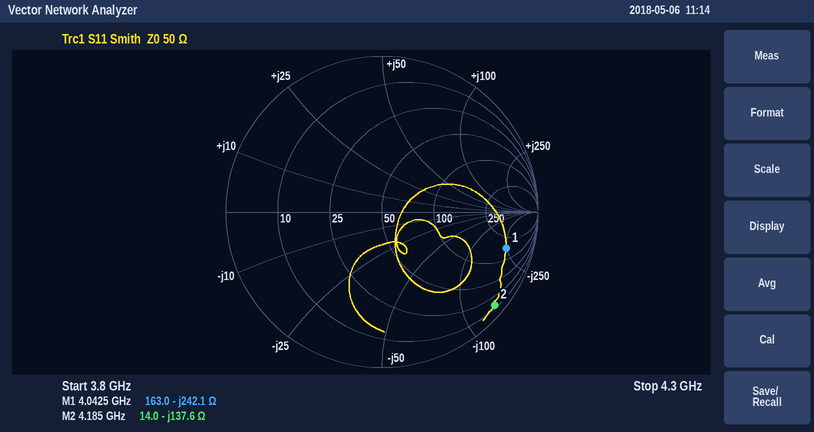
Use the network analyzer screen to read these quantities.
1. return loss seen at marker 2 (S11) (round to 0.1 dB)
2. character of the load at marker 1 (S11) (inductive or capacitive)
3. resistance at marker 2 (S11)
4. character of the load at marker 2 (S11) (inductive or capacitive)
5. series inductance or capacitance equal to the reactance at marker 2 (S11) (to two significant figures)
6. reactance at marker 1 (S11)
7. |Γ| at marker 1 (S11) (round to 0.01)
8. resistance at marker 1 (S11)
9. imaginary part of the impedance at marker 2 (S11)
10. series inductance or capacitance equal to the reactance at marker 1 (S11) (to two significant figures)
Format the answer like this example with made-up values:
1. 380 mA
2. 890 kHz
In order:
1. 0.6 dB
2. capacitive
3. 14.0 Ω
4. capacitive
5. 280 fF
6. -242.1 Ω
7. 0.83
8. 163.0 Ω
9. -137.6 Ω
10. 160 fF
